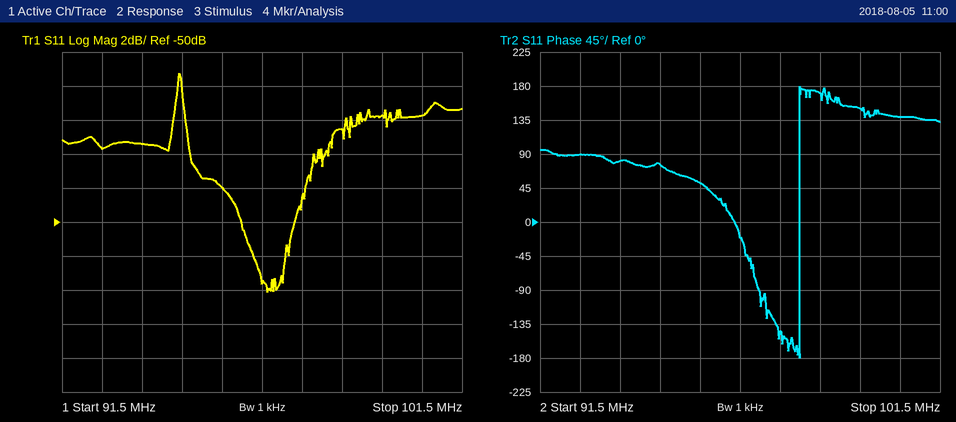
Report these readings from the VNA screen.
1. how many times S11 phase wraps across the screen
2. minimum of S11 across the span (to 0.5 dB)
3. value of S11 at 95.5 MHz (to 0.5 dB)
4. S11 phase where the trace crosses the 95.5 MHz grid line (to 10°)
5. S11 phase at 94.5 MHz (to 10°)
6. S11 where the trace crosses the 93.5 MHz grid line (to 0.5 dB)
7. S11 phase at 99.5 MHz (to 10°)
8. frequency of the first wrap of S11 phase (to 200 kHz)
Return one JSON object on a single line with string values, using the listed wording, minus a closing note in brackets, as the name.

{"how many times S11 phase wraps across the screen": "1", "minimum of S11 across the span": "-54.0 dB", "value of S11 at 95.5 MHz": "-48.0 dB", "S11 phase where the trace crosses the 95.5 MHz grid line": "50°", "S11 phase at 94.5 MHz": "80°", "S11 where the trace crosses the 93.5 MHz grid line": "-45.5 dB", "S11 phase at 99.5 MHz": "150°", "frequency of the first wrap of S11 phase": "98.0 MHz"}
